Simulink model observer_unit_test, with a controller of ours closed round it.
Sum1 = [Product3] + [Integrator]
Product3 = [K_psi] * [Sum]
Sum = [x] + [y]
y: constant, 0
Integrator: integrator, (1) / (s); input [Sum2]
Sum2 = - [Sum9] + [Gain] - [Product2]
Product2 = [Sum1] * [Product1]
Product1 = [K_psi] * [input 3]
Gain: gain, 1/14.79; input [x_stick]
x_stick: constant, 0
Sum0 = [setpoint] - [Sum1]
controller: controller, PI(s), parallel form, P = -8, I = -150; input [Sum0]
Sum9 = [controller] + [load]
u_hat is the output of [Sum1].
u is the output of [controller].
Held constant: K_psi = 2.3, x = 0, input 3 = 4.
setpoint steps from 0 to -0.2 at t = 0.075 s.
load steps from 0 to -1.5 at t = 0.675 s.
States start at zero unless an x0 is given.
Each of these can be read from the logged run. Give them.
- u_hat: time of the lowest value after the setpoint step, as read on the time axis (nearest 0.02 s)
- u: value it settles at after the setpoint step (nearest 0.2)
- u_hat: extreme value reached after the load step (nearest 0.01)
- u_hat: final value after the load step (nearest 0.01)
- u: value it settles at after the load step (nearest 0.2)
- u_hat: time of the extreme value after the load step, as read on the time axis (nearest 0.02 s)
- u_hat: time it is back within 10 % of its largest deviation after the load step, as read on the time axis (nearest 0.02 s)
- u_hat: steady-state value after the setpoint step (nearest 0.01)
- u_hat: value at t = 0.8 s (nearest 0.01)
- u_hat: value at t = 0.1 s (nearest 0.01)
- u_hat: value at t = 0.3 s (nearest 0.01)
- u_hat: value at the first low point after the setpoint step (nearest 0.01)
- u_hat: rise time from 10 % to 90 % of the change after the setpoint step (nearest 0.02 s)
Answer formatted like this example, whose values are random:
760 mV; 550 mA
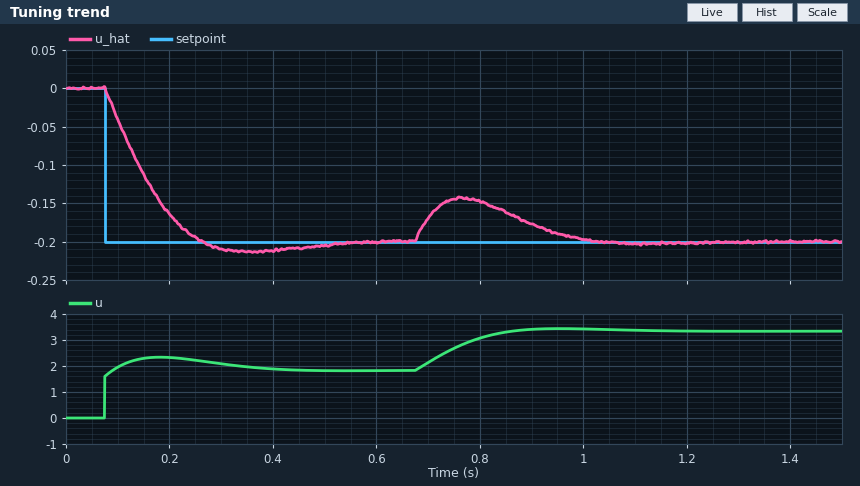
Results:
0.36 s; 1.8; -0.14; -0.20; 3.4; 0.76 s; 0.98 s; -0.20; -0.15; -0.04; -0.21; -0.21; 0.14 s
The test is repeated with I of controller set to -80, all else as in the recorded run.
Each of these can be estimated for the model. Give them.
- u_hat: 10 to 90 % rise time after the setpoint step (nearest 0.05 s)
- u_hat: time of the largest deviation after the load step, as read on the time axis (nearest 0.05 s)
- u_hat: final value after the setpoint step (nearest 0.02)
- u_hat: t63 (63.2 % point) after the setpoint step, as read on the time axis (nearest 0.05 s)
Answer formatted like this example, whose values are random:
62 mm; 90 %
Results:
0.25 s; 0.80 s; -0.20; 0.20 s
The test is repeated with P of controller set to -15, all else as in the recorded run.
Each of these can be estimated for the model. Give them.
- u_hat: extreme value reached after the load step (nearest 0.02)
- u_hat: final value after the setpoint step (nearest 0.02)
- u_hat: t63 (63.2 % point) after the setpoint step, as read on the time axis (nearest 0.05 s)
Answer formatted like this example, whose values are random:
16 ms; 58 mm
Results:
-0.16; -0.20; 0.15 s
